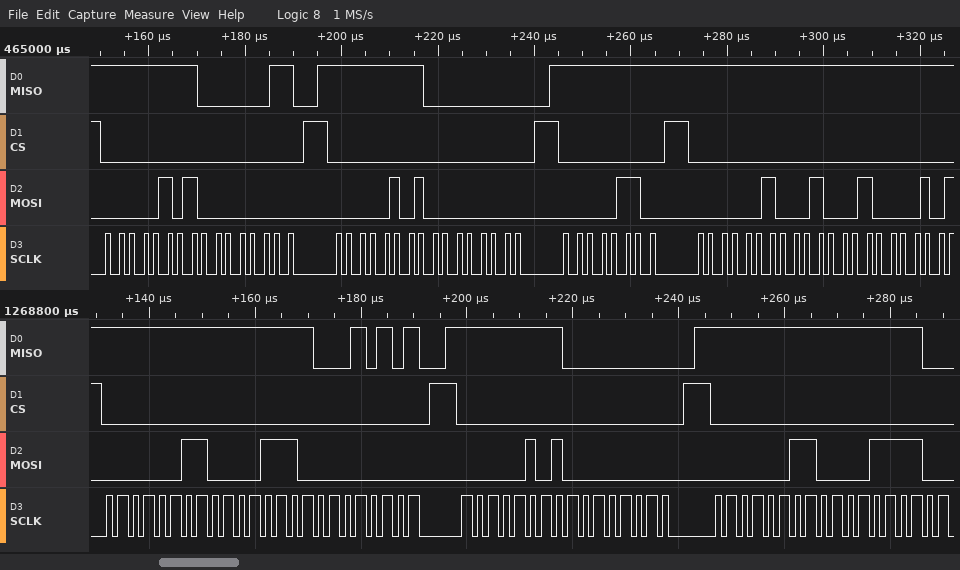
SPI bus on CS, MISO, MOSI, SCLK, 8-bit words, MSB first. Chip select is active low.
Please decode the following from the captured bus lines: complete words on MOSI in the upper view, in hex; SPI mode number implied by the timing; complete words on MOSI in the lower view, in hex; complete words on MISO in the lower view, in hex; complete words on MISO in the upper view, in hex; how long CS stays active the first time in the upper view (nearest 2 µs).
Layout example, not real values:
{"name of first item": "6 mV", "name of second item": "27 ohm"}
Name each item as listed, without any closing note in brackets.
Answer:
{"complete words on MOSI in the upper view, in hex": "05, 00, 05, 00, 06, 02, 22", "SPI mode number implied by the timing": "0", "complete words on MOSI in the lower view, in hex": "03, 0E, 00, 05, 00, 03, 0F", "complete words on MISO in the lower view, in hex": "FF, FF, 15, FF, 00, FF, FF", "complete words on MISO in the upper view, in hex": "FF, 03, FF, 00, FF, FF, FF", "how long CS stays active the first time in the upper view": "42 µs"}
